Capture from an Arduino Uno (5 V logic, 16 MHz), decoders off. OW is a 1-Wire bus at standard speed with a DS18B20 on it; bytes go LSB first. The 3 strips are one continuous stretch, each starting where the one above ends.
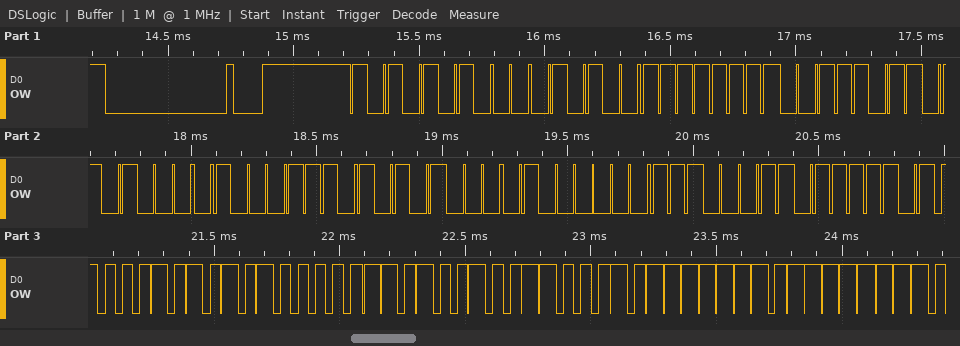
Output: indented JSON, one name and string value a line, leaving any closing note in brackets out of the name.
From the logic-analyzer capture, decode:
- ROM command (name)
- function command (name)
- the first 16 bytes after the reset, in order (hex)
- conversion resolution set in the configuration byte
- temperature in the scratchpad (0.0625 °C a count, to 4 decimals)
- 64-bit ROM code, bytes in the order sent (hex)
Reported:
{
  "ROM command": "Match ROM",
  "function command": "Read Scratchpad",
  "the first 16 bytes after the reset, in order": "55 28 FF DC 0A 71 15 02 C7 BE 50 05 4B 46 7F FF",
  "conversion resolution set in the configuration byte": "12 bits",
  "temperature in the scratchpad": "85.0000 °C",
  "64-bit ROM code, bytes in the order sent": "28 FF DC 0A 71 15 02 C7"
}
